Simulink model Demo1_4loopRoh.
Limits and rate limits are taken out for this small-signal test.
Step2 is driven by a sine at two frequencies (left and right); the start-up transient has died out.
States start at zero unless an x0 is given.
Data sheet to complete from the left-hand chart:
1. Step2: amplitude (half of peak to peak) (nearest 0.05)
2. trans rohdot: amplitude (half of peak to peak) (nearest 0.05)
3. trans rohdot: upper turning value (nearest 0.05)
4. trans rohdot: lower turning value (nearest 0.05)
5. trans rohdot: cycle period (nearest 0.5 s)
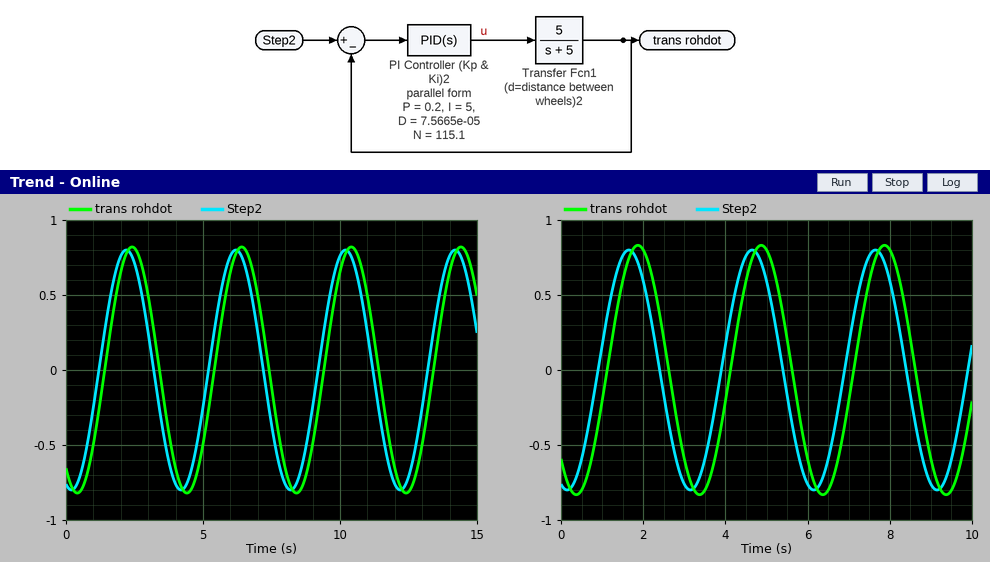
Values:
0.80
0.80
0.80
-0.80
4.0 s
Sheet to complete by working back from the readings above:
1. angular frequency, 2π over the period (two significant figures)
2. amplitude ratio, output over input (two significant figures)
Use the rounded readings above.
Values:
1.6 rad/s
1.0
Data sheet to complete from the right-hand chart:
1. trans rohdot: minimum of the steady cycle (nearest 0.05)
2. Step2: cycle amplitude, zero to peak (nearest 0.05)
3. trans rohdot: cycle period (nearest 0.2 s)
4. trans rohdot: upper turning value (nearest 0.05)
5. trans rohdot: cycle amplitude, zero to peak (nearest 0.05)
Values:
-0.85
0.80
3.0 s
0.85
0.85
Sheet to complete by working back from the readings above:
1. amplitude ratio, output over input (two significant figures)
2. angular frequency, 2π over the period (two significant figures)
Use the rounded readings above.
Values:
1.1
2.1 rad/s
